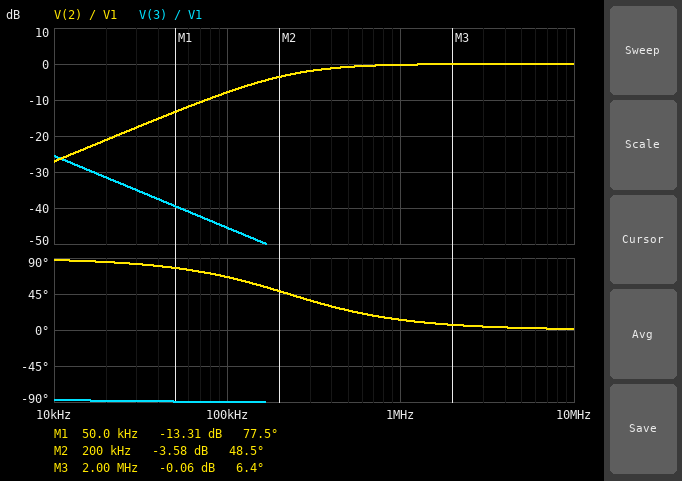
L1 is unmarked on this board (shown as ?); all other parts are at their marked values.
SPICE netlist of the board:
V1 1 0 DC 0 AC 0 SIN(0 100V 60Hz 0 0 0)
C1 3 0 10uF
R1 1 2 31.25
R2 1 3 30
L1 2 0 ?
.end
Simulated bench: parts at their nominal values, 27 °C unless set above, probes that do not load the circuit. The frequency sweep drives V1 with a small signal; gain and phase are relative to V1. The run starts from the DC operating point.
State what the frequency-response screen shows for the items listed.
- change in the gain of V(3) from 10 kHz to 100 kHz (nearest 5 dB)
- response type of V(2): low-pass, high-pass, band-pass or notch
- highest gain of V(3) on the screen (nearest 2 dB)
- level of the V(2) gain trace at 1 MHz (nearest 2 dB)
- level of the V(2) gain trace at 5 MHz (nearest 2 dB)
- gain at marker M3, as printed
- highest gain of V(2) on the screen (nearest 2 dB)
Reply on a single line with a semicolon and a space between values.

-20 dB; high-pass; -26 dB; 0 dB; 0 dB; -0.06 dB; 0 dB
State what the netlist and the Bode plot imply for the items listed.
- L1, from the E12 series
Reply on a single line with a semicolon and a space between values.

22 µH
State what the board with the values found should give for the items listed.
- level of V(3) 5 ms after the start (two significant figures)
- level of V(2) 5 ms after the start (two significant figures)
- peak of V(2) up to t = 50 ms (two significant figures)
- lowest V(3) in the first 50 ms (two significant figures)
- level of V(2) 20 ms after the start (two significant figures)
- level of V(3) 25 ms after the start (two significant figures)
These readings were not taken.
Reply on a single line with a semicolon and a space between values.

97 V; -8.2 mV; 27 mV; -99 V; 8.2 mV; 11 V
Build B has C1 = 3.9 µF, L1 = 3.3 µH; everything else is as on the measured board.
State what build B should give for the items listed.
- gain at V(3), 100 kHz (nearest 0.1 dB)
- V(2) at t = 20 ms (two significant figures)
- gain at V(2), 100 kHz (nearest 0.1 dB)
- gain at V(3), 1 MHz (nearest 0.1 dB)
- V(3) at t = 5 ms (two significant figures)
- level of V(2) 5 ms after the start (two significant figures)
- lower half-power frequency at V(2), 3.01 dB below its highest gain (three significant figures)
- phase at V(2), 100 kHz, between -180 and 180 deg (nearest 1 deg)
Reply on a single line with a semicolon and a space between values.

-37.3 dB; 1.2 mV; -23.6 dB; -57.3 dB; 96 V; -1.2 mV; 1.51 MHz; 86 deg
